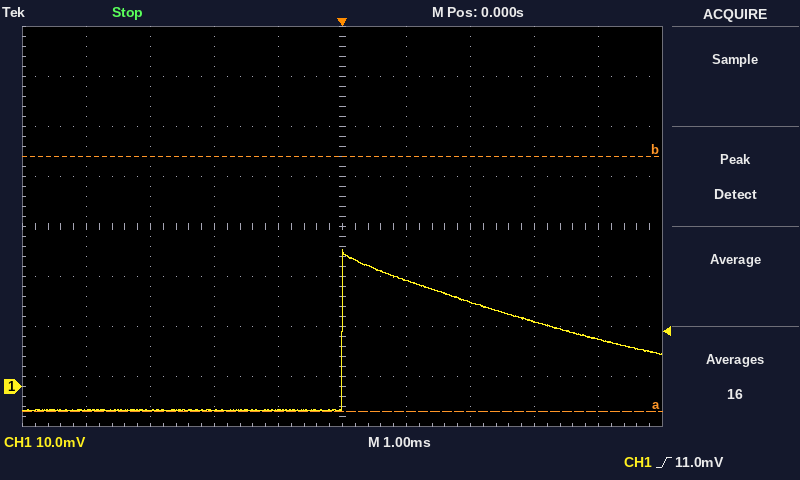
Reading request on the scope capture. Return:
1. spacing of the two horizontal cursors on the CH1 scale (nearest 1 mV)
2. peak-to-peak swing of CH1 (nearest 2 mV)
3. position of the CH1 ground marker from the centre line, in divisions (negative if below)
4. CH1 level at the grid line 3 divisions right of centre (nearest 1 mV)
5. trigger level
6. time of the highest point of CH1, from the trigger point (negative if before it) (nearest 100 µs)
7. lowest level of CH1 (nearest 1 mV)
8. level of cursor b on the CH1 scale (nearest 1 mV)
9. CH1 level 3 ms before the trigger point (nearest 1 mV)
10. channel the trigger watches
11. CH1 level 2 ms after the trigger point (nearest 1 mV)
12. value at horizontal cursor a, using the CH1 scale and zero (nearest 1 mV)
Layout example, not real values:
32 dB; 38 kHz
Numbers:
51 mV; 32 mV; -3.2 div; 13 mV; 11.0 mV; 0.0 ms; -5 mV; 46 mV; -5 mV; CH1; 17 mV; -5 mV
